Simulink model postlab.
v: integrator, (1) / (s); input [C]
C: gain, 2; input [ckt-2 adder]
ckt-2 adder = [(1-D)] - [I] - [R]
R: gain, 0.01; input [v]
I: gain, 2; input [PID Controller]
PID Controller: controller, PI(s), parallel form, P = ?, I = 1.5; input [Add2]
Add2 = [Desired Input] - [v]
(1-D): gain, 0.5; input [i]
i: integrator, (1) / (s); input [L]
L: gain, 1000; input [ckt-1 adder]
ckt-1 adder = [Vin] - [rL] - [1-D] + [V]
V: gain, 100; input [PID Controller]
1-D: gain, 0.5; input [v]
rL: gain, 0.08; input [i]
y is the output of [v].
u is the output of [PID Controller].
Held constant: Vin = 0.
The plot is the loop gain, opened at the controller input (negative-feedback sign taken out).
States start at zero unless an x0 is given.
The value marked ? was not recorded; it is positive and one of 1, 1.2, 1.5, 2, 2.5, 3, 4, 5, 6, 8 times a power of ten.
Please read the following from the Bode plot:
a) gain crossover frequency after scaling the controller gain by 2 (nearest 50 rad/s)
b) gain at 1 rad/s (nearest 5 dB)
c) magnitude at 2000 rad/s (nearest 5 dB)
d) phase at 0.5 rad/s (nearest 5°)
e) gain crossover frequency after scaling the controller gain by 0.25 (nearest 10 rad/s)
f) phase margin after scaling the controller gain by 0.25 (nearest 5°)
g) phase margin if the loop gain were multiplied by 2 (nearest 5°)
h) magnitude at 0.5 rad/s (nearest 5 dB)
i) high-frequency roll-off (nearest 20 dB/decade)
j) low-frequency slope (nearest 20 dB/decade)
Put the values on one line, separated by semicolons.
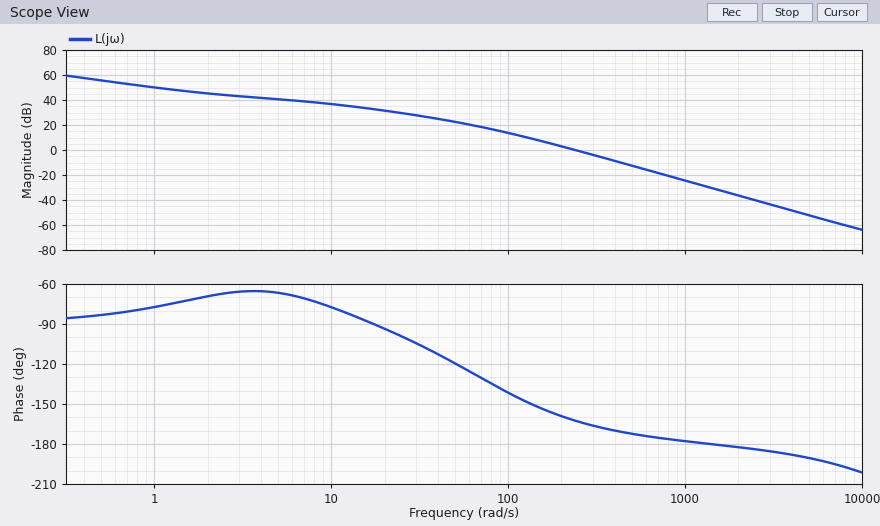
350 rad/s; 50 dB; -35 dB; -85°; 110 rad/s; 35°; 10°; 55 dB; -40 dB/decade; -20 dB/decade
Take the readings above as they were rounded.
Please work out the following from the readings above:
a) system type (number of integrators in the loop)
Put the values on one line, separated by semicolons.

1
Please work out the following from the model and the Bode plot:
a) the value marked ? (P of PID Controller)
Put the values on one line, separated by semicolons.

0.6
